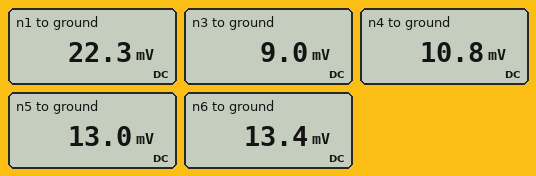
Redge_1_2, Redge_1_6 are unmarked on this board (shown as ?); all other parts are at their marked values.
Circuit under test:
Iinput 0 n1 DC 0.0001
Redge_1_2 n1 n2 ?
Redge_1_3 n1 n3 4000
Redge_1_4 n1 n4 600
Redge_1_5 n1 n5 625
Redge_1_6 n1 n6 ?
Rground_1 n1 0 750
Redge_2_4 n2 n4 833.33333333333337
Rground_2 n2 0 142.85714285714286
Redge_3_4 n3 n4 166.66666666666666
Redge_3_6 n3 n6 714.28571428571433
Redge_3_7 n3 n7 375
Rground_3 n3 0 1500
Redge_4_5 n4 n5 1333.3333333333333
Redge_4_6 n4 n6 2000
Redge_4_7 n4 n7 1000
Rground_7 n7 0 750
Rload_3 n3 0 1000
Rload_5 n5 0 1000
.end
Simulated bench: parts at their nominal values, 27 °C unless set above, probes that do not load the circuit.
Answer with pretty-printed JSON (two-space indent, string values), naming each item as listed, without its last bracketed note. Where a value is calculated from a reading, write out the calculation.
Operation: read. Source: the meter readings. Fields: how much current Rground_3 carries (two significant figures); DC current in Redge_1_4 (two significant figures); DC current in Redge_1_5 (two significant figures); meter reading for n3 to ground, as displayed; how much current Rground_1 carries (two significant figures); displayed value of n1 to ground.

{
  "how much current Rground_3 carries": "(9 mV) / 1.5 kΩ = 6.0 µA",
  "DC current in Redge_1_4": "(22.3 mV - 10.8 mV) / 600 Ω = 19 µA",
  "DC current in Redge_1_5": "(22.3 mV - 13 mV) / 625 Ω = 15 µA",
  "meter reading for n3 to ground, as displayed": "9.0 mV",
  "how much current Rground_1 carries": "(22.3 mV) / 750 Ω = 30 µA",
  "displayed value of n1 to ground": "22.3 mV"
}
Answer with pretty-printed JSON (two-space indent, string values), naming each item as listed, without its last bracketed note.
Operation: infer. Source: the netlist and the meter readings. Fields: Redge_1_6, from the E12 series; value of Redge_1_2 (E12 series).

{
  "Redge_1_6, from the E12 series": "1.2 kΩ",
  "value of Redge_1_2": "680 Ω"
}
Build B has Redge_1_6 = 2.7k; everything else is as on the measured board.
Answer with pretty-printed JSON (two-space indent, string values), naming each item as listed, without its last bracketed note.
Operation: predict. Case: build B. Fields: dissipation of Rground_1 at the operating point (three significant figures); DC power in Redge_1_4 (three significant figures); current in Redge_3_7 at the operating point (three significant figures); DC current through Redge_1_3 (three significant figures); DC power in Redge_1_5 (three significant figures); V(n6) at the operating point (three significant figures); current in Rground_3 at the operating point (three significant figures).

{
  "dissipation of Rground_1 at the operating point": "688 nW",
  "DC power in Redge_1_4": "247 nW",
  "current in Redge_3_7 at the operating point": "5.03 µA",
  "DC current through Redge_1_3": "3.54 µA",
  "DC power in Redge_1_5": "145 nW",
  "V(n6) at the operating point": "11.3 mV",
  "current in Rground_3 at the operating point": "5.70 µA"
}
